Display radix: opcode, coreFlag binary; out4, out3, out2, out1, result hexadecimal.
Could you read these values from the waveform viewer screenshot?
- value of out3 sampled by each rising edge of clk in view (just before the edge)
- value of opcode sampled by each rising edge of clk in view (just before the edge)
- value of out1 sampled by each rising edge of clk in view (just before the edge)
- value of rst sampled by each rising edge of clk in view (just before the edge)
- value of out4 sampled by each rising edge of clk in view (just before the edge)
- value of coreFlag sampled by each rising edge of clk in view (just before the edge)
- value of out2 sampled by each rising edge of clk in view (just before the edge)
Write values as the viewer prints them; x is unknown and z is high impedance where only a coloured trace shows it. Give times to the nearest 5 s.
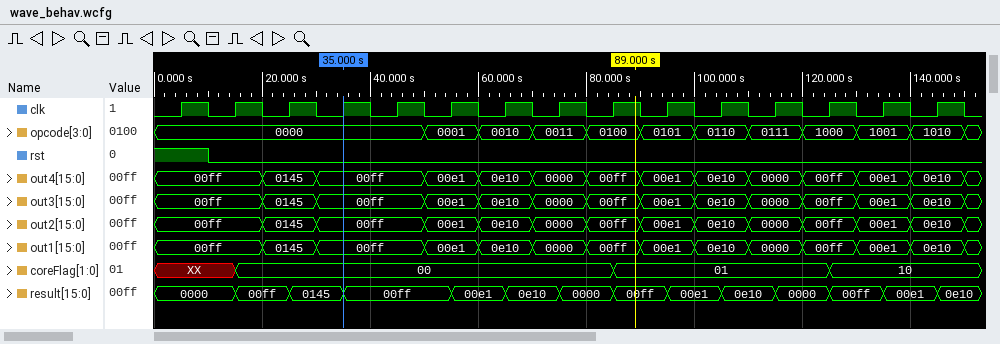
00ff, 00ff, 0145, 00ff, 00ff, 00e1, 0e10, 0000, 00ff, 00e1, 0e10, 0000, 00ff, 00e1, 0e10
0000, 0000, 0000, 0000, 0000, 0001, 0010, 0011, 0100, 0101, 0110, 0111, 1000, 1001, 1010
00ff, 00ff, 0145, 00ff, 00ff, 00e1, 0e10, 0000, 00ff, 00e1, 0e10, 0000, 00ff, 00e1, 0e10
1 0 0 0 0 0 0 0 0 0 0 0 0 0 0
00ff, 00ff, 0145, 00ff, 00ff, 00e1, 0e10, 0000, 00ff, 00e1, 0e10, 0000, 00ff, 00e1, 0e10
XX, XX, 00, 00, 00, 00, 00, 00, 00, 01, 01, 01, 01, 10, 10
00ff, 00ff, 0145, 00ff, 00ff, 00e1, 0e10, 0000, 00ff, 00e1, 0e10, 0000, 00ff, 00e1, 0e10
